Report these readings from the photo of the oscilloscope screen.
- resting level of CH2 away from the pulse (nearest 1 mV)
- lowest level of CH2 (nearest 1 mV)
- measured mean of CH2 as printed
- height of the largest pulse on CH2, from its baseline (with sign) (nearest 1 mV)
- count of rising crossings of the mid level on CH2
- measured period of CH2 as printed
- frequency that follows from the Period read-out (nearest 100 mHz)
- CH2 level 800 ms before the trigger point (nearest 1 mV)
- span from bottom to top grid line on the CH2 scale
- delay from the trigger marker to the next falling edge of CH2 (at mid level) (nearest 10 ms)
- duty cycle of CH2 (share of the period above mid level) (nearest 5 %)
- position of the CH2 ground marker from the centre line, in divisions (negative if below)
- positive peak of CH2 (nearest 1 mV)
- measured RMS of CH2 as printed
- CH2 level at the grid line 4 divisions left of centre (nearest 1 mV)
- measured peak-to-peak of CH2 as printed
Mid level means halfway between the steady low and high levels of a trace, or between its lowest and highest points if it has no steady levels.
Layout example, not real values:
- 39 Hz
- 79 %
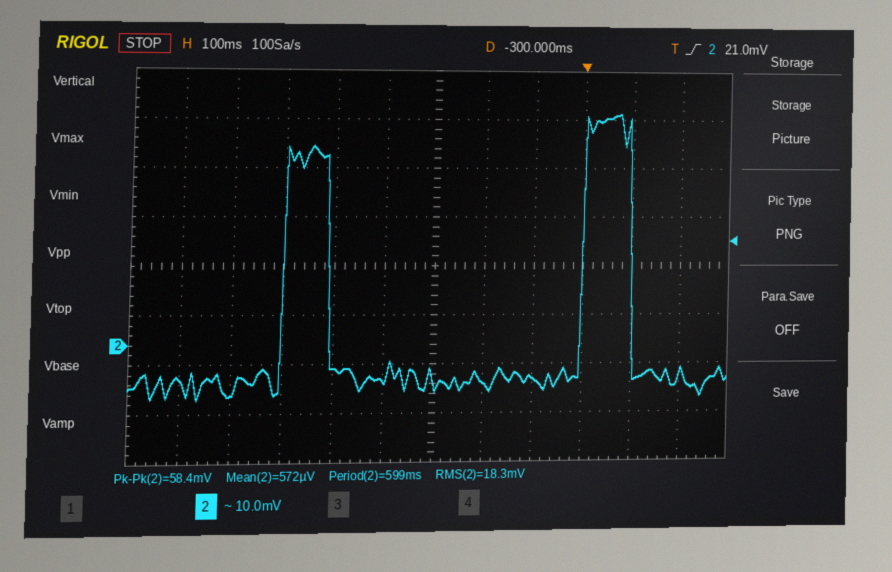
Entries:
- -7 mV
- -11 mV
- 572 µV
- +54 mV
- 2
- 599 ms
- 1.7 Hz
- -7 mV
- 80 mV
- 100 ms
- 15 %
- -1.6 div
- 47 mV
- 18.3 mV
- -10 mV
- 58.4 mV
